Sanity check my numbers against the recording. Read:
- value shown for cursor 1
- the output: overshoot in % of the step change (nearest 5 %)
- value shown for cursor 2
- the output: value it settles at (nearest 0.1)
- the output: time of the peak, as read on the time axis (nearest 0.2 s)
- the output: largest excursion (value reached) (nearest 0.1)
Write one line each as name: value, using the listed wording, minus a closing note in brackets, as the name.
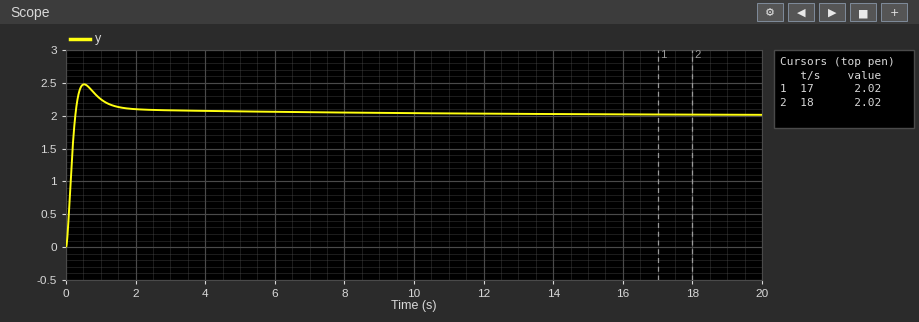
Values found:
value shown for cursor 1: 2.02
the output: overshoot in % of the step change: 25 %
value shown for cursor 2: 2.02
the output: value it settles at: 2.0
the output: time of the peak, as read on the time axis: 0.6 s
the output: largest excursion (value reached): 2.5
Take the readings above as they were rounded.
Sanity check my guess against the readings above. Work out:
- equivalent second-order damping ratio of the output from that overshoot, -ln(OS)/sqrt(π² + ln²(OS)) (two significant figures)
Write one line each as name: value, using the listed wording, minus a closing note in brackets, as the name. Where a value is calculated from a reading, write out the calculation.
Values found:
equivalent second-order damping ratio of the output from that overshoot, -ln(OS)/sqrt(π² + ln²(OS)): ln(0.25) = -1.386; 1.386 / sqrt(9.870 + 1.922) = 0.40
